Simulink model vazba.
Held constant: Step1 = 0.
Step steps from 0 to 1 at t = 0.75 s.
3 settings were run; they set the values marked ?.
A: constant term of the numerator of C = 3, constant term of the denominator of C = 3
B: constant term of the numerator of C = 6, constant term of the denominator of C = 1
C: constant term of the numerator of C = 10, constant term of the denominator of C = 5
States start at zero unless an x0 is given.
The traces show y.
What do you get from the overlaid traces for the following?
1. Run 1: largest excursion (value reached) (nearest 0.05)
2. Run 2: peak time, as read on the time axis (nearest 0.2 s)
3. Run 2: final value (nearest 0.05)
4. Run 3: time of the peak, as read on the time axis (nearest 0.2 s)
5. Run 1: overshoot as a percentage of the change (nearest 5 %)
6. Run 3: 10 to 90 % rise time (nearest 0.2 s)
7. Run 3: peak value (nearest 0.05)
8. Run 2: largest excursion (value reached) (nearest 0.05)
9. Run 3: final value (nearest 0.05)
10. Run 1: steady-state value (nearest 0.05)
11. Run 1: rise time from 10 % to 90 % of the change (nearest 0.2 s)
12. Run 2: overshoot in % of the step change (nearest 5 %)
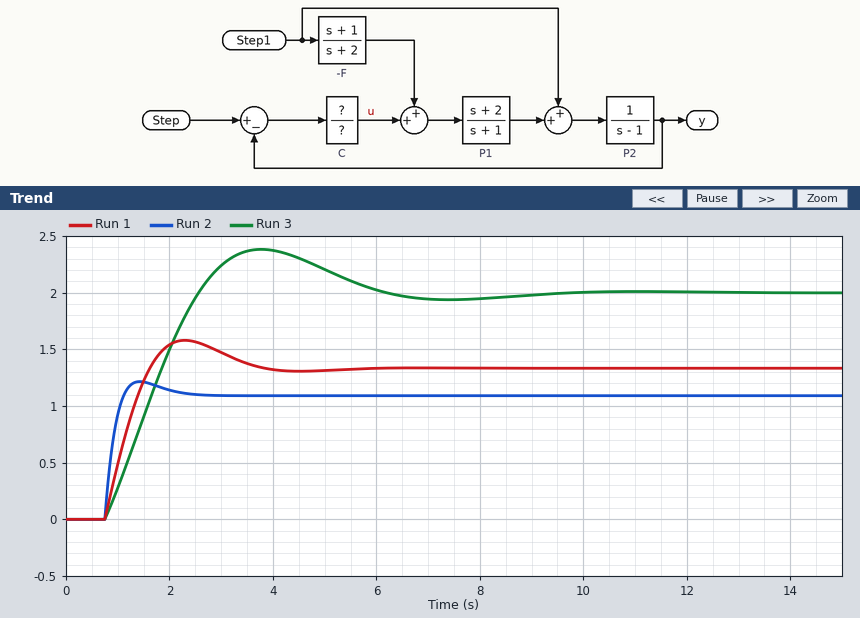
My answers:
1.60
1.4 s
1.10
3.8 s
20 %
1.4 s
2.40
1.20
2.00
1.35
0.6 s
10 %
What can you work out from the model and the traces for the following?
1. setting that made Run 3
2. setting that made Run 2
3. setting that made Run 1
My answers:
A
B
C
